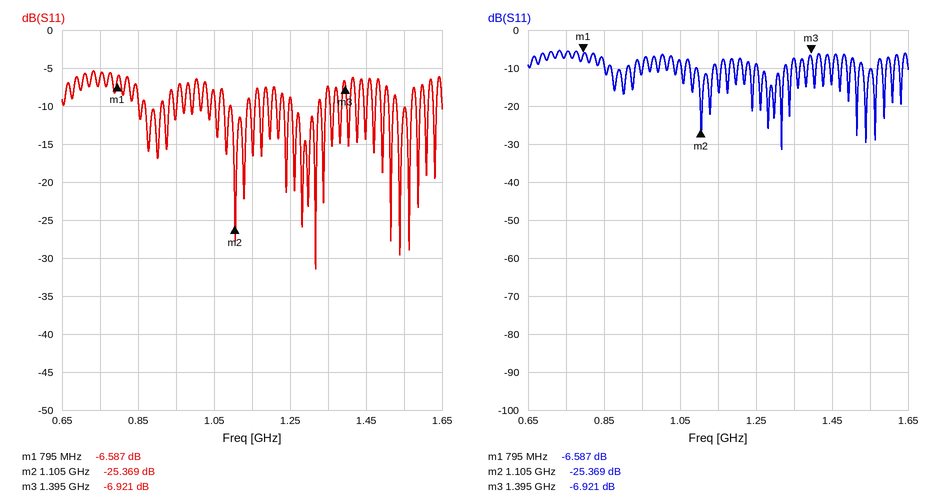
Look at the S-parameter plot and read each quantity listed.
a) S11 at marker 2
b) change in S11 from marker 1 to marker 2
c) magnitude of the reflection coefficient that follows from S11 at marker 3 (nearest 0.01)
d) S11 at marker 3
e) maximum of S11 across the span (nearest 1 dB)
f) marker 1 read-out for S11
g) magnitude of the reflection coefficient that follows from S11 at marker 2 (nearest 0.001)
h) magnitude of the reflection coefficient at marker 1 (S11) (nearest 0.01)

-25.369 dB
-18.782 dB
0.45
-6.921 dB
-5 dB
-6.587 dB
0.054
0.47
